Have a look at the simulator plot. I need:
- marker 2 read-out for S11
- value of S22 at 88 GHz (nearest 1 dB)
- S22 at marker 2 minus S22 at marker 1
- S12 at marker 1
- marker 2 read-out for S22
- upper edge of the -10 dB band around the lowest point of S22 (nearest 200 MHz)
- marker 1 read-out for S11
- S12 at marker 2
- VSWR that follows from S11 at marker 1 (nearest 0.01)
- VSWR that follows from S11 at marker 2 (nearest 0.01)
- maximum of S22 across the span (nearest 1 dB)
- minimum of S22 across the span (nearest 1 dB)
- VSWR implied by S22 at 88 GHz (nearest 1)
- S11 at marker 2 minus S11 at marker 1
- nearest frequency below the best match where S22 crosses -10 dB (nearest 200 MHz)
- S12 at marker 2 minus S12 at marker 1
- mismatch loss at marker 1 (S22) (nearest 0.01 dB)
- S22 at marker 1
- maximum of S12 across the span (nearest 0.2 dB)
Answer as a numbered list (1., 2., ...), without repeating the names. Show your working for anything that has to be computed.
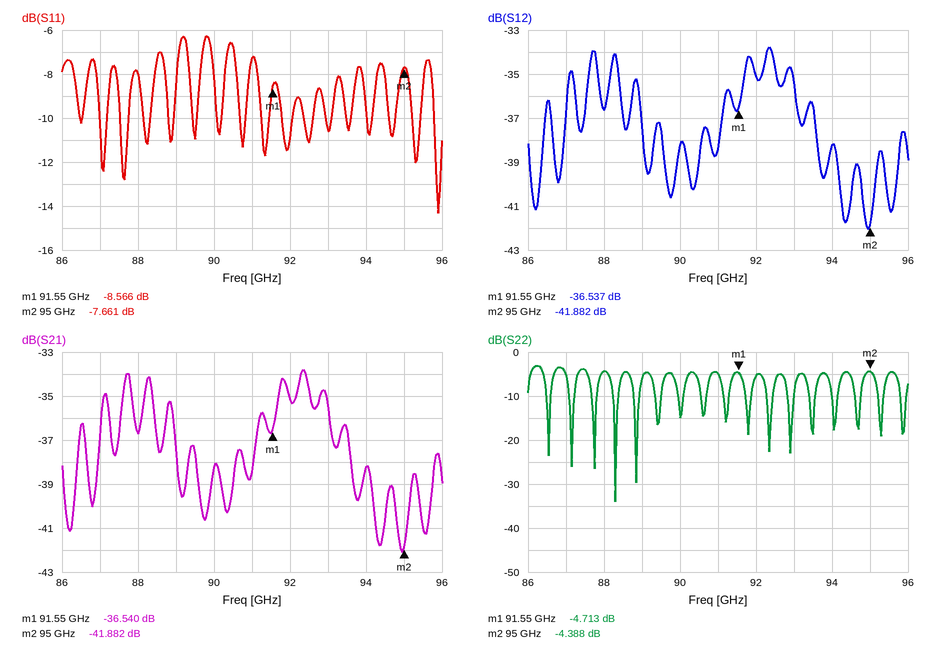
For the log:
1. -7.661 dB
2. -4 dB
3. -4.388 − (-4.713) = 0.325 dB
4. -36.537 dB
5. -4.388 dB
6. 88.4 GHz
7. -8.566 dB
8. -41.882 dB
9. (1 + 0.3730)/(1 − 0.3730) ≈ 2.19
10. (1 + 0.4140)/(1 − 0.4140) ≈ 2.41
11. -3 dB
12. -34 dB
13. |Γ| = 10^(-4/20) = 0.6310; VSWR = (1 + 0.6310)/(1 − 0.6310) ≈ 4
14. -7.661 − (-8.566) = 0.905 dB
15. 88.2 GHz
16. -41.882 − (-36.537) = -5.345 dB
17. −10 log10(1 − 10^(-4.713/10)) ≈ 1.79 dB
18. -4.713 dB
19. -33.8 dB
